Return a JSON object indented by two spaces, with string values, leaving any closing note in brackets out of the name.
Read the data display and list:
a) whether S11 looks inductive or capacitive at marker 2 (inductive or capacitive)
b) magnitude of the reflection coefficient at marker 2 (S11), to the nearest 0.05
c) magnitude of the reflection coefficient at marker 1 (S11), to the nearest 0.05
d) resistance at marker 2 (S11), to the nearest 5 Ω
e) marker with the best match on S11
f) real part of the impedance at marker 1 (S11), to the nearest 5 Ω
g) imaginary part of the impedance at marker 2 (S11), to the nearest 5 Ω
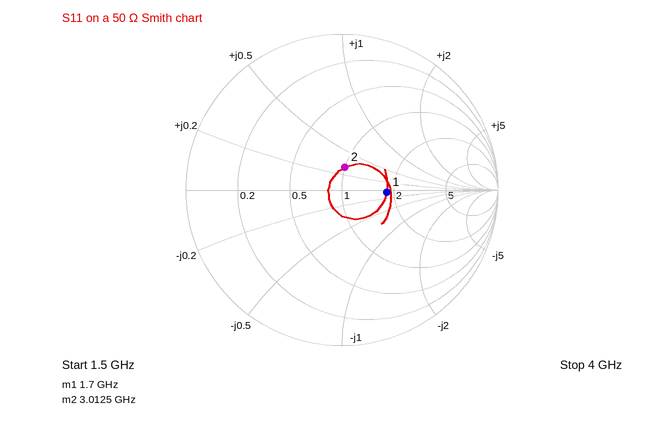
{
  "whether S11 looks inductive or capacitive at marker 2": "inductive",
  "magnitude of the reflection coefficient at marker 2 (S11), to the nearest 0.05": "0.15",
  "magnitude of the reflection coefficient at marker 1 (S11), to the nearest 0.05": "0.30",
  "resistance at marker 2 (S11), to the nearest 5 Ω": "50 Ω",
  "marker with the best match on S11": "marker 2",
  "real part of the impedance at marker 1 (S11), to the nearest 5 Ω": "90 Ω",
  "imaginary part of the impedance at marker 2 (S11), to the nearest 5 Ω": "+15 Ω"
}
